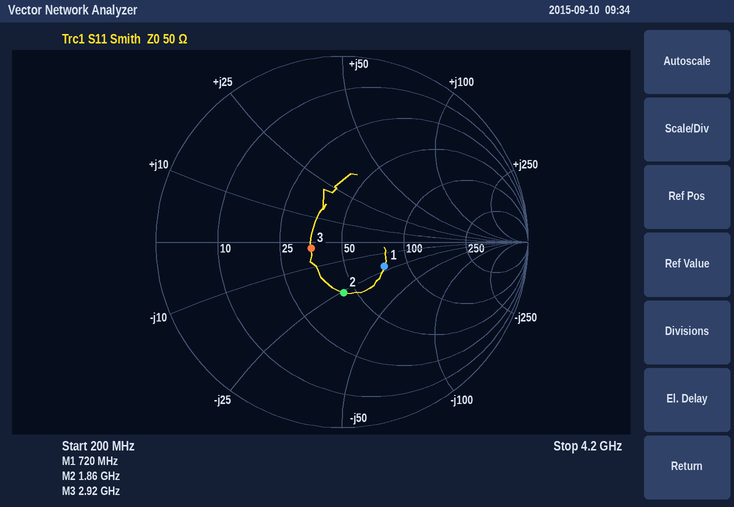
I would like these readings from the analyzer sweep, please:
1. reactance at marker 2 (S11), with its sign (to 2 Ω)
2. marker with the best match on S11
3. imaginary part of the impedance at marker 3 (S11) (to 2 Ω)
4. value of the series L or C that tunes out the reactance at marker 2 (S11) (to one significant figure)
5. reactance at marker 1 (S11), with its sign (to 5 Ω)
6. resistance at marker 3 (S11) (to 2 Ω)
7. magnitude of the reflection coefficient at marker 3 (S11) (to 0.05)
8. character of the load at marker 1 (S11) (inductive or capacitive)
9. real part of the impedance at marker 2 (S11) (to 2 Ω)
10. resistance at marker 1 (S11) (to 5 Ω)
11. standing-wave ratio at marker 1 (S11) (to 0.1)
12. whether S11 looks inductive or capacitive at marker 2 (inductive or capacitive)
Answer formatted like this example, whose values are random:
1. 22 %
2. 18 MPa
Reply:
1. -26 Ω
2. marker 3
3. -2 Ω
4. 2 nH
5. -20 Ω
6. 36 Ω
7. 0.15
8. capacitive
9. 44 Ω
10. 75 Ω
11. 1.7
12. capacitive
